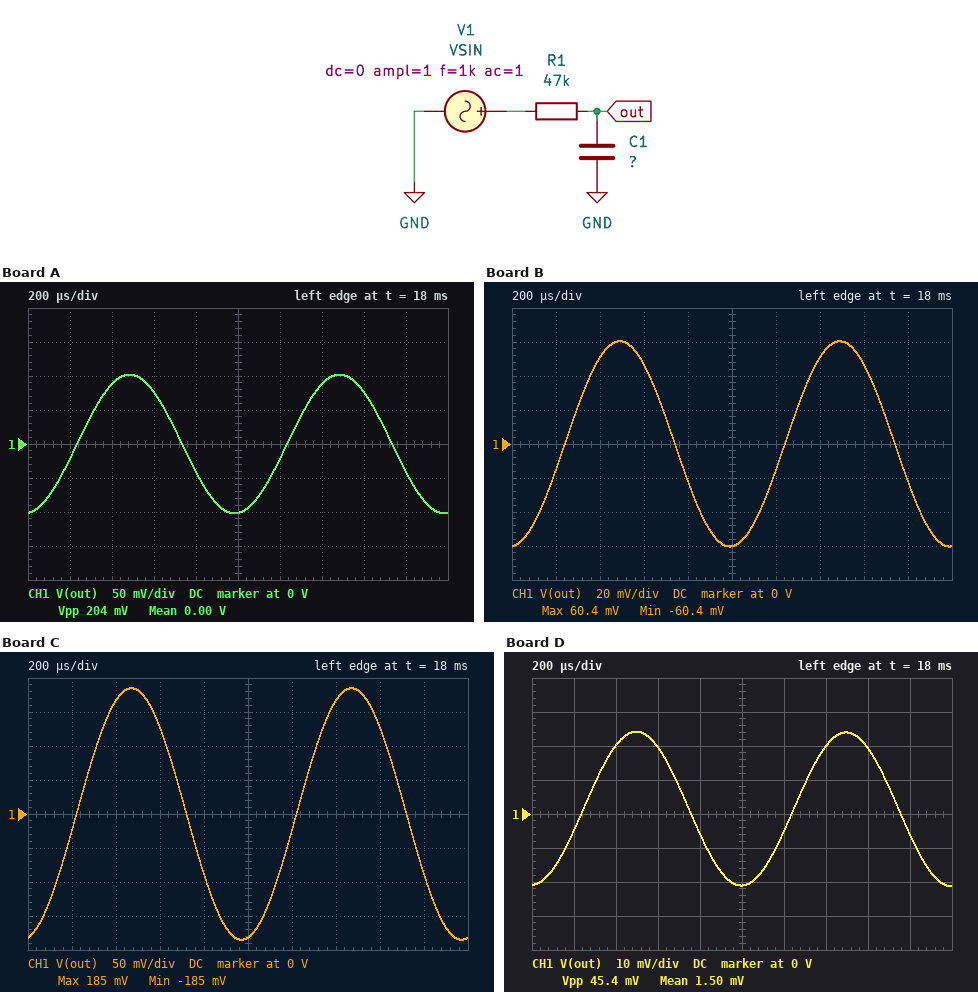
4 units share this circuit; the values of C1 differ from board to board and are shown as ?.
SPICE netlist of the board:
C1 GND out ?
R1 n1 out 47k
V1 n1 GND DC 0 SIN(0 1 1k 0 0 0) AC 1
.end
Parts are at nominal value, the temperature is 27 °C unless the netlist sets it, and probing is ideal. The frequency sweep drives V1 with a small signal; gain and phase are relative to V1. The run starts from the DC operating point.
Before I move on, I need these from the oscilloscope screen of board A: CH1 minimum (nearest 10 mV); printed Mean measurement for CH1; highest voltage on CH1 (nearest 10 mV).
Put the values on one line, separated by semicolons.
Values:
-100 mV; 0.00 V; 100 mV
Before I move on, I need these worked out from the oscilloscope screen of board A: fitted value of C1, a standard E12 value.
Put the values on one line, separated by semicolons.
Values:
33 nF
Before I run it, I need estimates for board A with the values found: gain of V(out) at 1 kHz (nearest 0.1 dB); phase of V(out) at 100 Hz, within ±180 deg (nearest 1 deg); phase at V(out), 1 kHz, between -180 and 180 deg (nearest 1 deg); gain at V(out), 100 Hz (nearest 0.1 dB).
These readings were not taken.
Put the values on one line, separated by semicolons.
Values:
-19.8 dB; -44 deg; -84 deg; -2.9 dB
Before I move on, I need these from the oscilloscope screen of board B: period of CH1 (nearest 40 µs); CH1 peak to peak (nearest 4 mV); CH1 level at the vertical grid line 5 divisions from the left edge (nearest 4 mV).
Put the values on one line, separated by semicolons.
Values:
1.00 ms; 120 mV; -60 mV
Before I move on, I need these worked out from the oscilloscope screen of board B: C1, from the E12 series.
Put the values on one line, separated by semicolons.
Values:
56 nF
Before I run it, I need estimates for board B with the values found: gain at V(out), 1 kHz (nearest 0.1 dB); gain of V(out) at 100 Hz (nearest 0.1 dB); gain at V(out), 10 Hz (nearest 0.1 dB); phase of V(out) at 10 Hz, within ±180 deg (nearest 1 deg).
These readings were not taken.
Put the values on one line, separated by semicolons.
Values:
-24.4 dB; -5.7 dB; -0.1 dB; -9 deg
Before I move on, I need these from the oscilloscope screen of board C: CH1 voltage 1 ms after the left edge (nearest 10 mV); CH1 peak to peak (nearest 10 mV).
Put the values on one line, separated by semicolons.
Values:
-180 mV; 370 mV
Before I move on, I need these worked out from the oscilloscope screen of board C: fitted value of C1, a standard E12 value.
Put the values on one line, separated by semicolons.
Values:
18 nF
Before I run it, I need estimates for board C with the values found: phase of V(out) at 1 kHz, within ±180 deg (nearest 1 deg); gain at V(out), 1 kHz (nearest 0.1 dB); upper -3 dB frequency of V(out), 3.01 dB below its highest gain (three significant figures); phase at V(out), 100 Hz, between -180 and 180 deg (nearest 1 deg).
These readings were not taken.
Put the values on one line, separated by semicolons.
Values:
-79 deg; -14.7 dB; 188 Hz; -28 deg
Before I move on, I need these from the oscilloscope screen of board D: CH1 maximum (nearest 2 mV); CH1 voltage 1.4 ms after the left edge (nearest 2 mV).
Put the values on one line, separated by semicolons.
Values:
24 mV; 20 mV
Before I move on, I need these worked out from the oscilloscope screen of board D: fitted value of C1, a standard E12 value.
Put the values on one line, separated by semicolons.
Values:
150 nF
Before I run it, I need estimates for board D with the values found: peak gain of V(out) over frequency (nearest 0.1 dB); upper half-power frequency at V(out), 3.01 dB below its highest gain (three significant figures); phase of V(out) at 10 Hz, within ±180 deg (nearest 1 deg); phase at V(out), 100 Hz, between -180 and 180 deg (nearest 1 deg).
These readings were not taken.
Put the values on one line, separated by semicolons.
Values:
0 dB; 22.6 Hz; -24 deg; -77 deg
